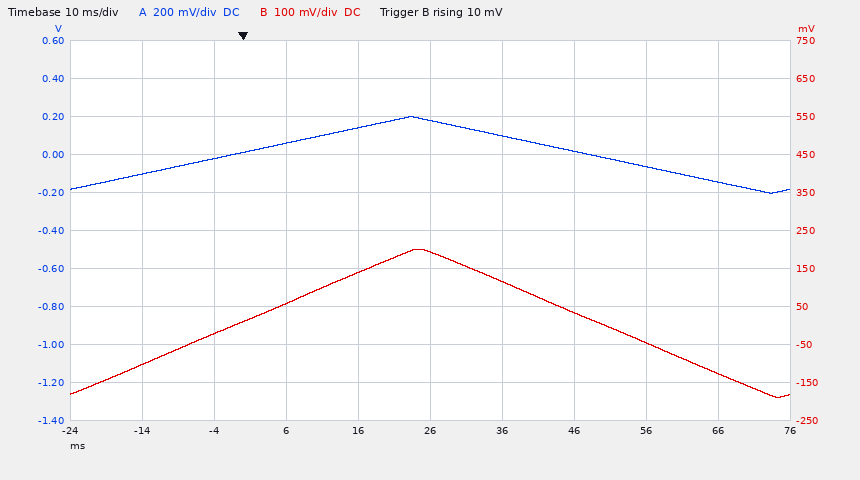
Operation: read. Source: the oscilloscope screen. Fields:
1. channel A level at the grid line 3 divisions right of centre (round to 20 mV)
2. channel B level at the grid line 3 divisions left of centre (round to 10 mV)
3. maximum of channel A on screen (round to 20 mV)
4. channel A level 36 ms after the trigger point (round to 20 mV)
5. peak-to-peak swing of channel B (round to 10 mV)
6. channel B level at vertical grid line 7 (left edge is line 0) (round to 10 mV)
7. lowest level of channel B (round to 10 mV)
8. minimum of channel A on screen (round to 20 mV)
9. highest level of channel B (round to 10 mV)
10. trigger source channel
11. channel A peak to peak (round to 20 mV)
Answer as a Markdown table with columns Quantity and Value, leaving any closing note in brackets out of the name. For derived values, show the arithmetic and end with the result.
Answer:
| Quantity | Value |
|---|---|
| channel A level at the grid line 3 divisions right of centre | -60 mV |
| channel B level at the grid line 3 divisions left of centre | -20 mV |
| maximum of channel A on screen | 200 mV |
| channel A level 36 ms after the trigger point | 100 mV |
| peak-to-peak swing of channel B | 200 mV − (-190 mV) = 390 mV |
| channel B level at vertical grid line 7 (left edge is line 0) | 30 mV |
| lowest level of channel B | -190 mV |
| minimum of channel A on screen | -200 mV |
| highest level of channel B | 200 mV |
| trigger source channel | channel B |
| channel A peak to peak | 200 mV − (-200 mV) = 400 mV |
